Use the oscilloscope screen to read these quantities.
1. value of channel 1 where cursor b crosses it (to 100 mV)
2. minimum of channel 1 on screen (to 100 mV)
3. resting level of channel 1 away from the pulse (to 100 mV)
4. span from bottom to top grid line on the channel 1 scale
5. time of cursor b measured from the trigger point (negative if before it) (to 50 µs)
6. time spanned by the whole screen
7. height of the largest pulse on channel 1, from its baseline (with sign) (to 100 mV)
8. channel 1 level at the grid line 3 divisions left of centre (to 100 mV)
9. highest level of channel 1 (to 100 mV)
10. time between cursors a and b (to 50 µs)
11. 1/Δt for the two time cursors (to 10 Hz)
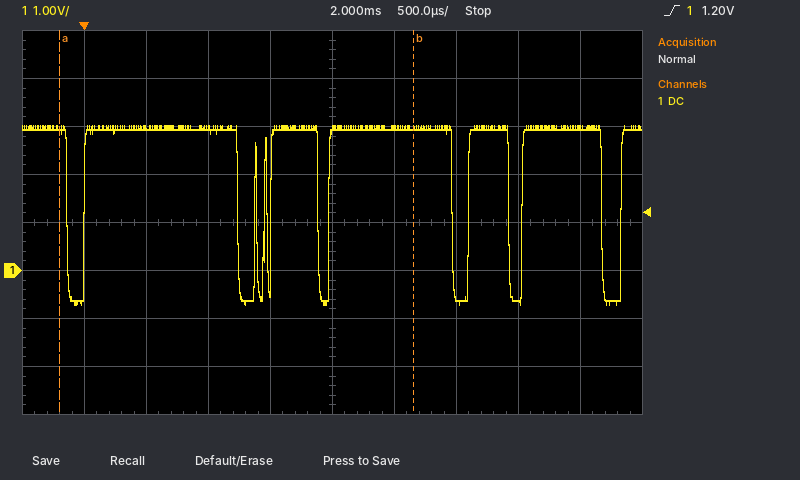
3.0 V
-700 mV
3.0 V
8 V
+2.65 ms
5 ms
-3.7 V
3.0 V
3.0 V
2.85 ms
350 Hz
